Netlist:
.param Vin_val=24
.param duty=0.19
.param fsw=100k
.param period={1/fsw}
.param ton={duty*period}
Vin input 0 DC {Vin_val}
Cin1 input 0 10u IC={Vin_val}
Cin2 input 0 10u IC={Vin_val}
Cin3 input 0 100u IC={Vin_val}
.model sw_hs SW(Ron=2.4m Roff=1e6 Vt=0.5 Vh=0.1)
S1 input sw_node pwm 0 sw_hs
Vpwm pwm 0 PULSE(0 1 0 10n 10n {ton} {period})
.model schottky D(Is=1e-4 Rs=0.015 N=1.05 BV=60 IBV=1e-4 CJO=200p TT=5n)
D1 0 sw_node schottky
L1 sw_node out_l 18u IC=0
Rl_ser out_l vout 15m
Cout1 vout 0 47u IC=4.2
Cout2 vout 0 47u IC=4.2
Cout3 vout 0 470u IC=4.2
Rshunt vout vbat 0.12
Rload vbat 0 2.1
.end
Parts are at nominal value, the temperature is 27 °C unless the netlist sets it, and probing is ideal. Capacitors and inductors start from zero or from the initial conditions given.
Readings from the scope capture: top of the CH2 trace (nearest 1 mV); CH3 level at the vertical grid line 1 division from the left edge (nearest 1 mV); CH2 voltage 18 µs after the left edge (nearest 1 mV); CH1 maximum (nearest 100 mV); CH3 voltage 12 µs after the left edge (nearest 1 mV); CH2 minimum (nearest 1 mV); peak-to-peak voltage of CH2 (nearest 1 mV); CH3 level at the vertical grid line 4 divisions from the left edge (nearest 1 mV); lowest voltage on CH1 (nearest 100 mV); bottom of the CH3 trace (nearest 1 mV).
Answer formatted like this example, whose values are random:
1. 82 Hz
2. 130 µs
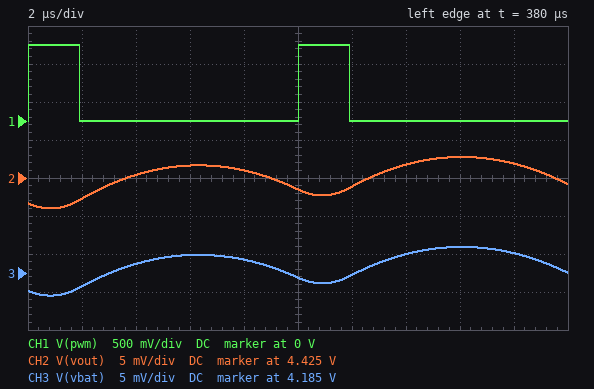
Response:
1. 4.428 V
2. 4.183 V
3. 4.427 V
4. 1.0 V
5. 4.185 V
6. 4.421 V
7. 7 mV
8. 4.187 V
9. 0 V
10. 4.182 V
